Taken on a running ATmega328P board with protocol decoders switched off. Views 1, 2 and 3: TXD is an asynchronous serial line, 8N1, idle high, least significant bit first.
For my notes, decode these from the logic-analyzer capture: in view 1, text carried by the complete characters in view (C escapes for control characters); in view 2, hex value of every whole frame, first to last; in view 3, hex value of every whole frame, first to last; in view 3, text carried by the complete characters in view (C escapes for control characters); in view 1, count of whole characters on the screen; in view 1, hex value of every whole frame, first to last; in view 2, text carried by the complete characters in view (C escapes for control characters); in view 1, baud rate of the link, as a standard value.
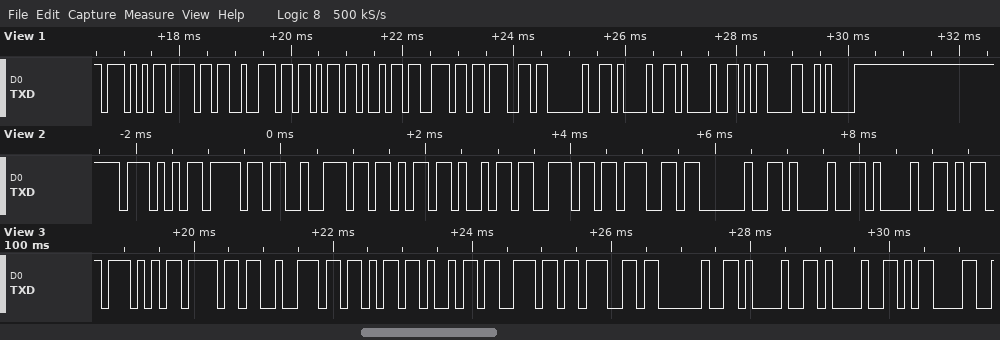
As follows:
"Working !!\r\n"
57 6F 72 6B 69 6E 67 20 21 21
57 6F 72 6B 69 6E 67 20 21 21 0D
"Working !!\r"
12
57 6F 72 6B 69 6E 67 20 21 21 0D 0A
"Working !!"
9600 baud
